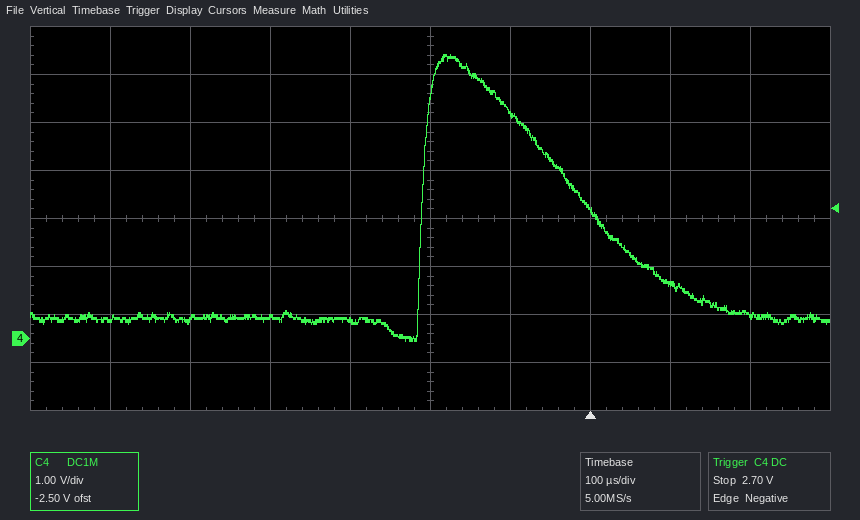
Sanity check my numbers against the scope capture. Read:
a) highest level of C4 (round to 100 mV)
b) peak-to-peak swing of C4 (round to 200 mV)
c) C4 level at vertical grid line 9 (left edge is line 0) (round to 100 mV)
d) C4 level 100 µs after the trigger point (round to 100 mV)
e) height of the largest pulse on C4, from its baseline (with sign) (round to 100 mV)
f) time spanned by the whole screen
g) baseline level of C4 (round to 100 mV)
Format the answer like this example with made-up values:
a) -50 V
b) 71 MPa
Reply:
a) 5.9 V
b) 6.0 V
c) 500 mV
d) 1.2 V
e) +5.5 V
f) 1 ms
g) 400 mV
